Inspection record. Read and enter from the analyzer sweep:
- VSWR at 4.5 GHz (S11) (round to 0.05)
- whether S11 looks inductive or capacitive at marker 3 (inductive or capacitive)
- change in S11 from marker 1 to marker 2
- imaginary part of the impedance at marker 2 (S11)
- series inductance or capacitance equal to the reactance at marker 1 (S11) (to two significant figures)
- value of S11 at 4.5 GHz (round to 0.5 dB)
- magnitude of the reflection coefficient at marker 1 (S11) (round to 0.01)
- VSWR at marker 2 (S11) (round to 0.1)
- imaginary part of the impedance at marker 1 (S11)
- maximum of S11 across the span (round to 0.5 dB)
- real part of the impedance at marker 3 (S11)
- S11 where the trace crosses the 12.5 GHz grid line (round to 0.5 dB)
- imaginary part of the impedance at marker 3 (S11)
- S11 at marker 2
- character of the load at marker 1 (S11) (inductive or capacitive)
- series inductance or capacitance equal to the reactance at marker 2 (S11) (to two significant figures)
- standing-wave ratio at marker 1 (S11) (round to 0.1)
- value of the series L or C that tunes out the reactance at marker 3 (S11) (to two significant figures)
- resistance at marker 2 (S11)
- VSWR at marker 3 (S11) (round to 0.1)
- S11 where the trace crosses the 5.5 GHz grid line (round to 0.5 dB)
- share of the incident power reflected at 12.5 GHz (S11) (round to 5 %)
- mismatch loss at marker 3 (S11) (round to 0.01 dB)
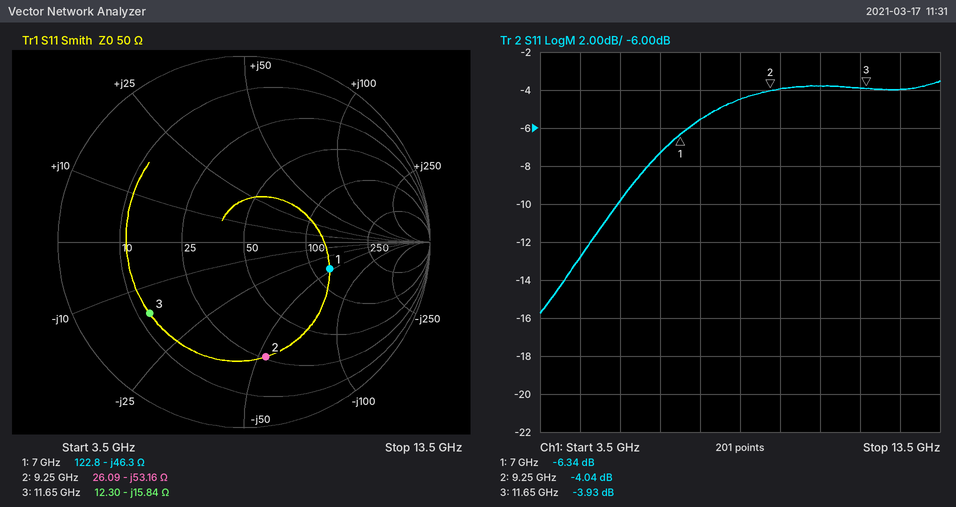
1.60
capacitive
2.30 dB
-53.16 Ω
490 fF
-13.0 dB
0.48
4.4
-46.3 Ω
-3.5 dB
12.30 Ω
-4.0 dB
-15.84 Ω
-4.04 dB
capacitive
320 fF
2.9
220 pH
26.09 Ω
4.5
-10.0 dB
40 %
2.25 dB
